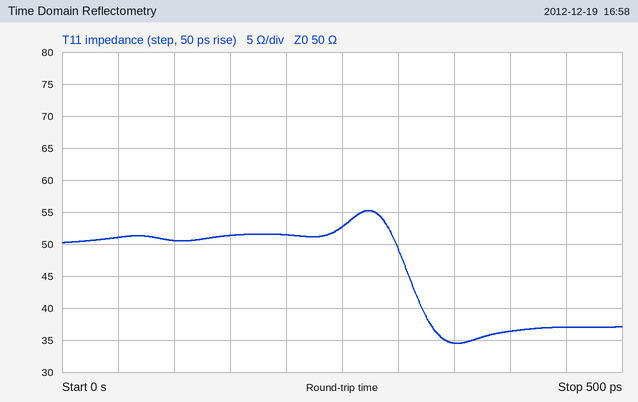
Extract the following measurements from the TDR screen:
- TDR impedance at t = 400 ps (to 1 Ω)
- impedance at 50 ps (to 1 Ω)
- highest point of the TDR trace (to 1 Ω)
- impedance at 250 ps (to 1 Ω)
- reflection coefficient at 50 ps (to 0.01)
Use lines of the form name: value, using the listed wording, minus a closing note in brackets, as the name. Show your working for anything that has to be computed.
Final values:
TDR impedance at t = 400 ps: 36 Ω
impedance at 50 ps: 51 Ω
highest point of the TDR trace: 55 Ω
impedance at 250 ps: 53 Ω
reflection coefficient at 50 ps: (51 − 50)/(51 + 50) ≈ +0.01
